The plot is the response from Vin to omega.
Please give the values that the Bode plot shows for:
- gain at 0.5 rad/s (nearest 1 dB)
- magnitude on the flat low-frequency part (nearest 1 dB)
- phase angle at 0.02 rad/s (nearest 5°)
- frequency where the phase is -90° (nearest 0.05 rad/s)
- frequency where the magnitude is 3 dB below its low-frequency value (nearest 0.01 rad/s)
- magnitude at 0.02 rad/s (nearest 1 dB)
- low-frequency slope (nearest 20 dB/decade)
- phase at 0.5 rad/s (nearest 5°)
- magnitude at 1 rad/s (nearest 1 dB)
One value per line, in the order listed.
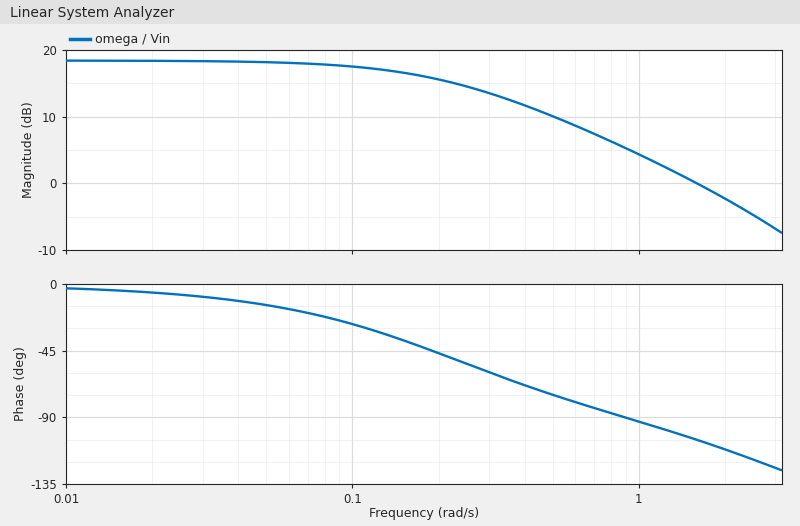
10 dB
18 dB
-5°
0.90 rad/s
0.21 rad/s
18 dB
0 dB/decade
-75°
4 dB
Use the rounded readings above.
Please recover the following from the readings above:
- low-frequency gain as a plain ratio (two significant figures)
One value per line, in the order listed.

7.9
